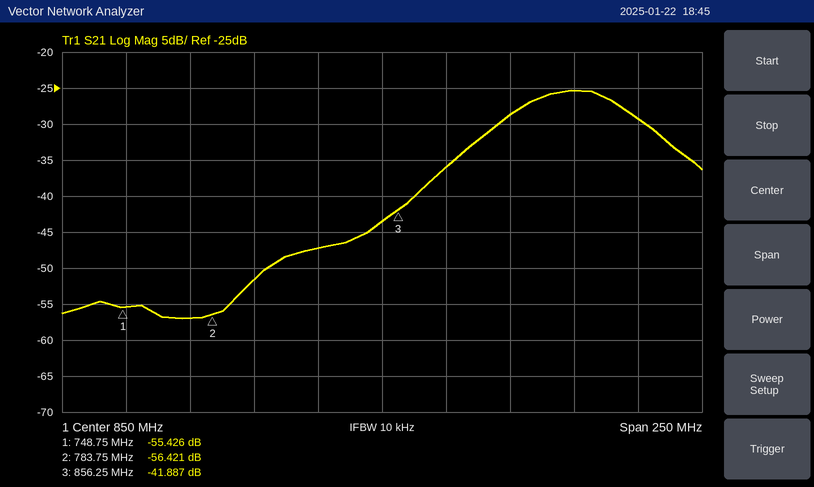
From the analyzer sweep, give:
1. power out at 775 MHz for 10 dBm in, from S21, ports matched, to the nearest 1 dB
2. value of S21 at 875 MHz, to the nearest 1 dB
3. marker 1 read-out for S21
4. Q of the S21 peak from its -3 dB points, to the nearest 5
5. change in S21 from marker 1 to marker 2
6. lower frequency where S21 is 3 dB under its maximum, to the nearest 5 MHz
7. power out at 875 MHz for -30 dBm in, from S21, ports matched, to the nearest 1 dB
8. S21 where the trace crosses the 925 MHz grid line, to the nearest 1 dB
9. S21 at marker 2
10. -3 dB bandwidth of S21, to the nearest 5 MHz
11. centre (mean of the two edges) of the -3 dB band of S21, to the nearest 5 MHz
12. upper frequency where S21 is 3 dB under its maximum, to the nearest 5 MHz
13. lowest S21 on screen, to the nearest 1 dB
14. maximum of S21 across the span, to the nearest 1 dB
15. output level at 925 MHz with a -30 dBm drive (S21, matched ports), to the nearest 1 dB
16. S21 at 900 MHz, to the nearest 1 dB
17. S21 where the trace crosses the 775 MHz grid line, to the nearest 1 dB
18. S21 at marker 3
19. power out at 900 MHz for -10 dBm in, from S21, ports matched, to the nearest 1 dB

-47 dBm
-36 dB
-55.426 dB
20
-0.995 dB
900 MHz
-66 dBm
-25 dB
-56.421 dB
45 MHz
925 MHz
945 MHz
-57 dB
-25 dB
-55 dBm
-29 dB
-57 dB
-41.887 dB
-39 dBm
